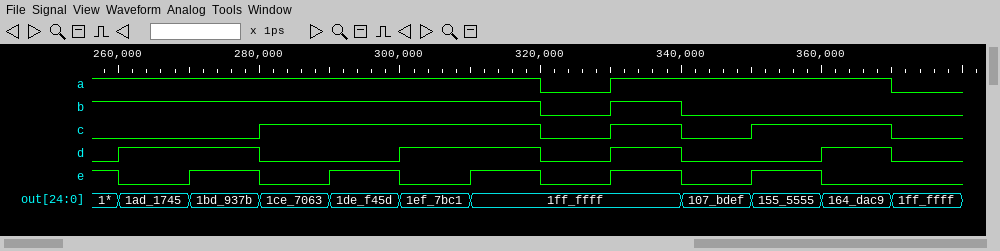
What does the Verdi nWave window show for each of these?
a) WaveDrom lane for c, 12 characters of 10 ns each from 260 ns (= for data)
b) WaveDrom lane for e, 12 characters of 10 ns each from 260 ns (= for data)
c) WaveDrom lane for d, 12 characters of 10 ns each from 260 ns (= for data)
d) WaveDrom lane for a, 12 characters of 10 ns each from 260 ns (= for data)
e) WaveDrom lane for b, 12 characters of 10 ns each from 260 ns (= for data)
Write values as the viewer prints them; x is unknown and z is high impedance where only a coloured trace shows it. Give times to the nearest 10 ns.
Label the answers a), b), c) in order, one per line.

a) {name: 'c', wave: '0.1...0101.0'}
b) {name: 'e', wave: '01010101010.'}
c) {name: 'd', wave: '1.0.1.010.10'}
d) {name: 'a', wave: '1.....01...0'}
e) {name: 'b', wave: '1.....010...'}
